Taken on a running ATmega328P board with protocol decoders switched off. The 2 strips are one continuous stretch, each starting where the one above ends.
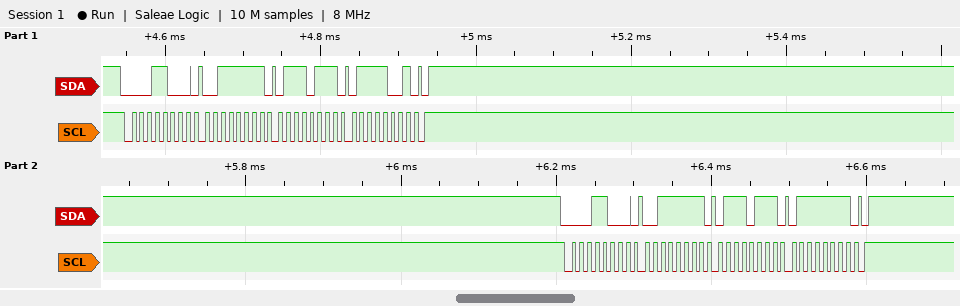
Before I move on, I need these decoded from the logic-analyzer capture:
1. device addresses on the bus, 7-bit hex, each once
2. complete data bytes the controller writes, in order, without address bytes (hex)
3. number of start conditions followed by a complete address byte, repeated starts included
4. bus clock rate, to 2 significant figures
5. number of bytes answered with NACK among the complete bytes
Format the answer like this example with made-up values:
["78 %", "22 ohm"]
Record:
["0x0C", "3F 77 79 3F 77 7F", "2", "100 kHz", "0"]
